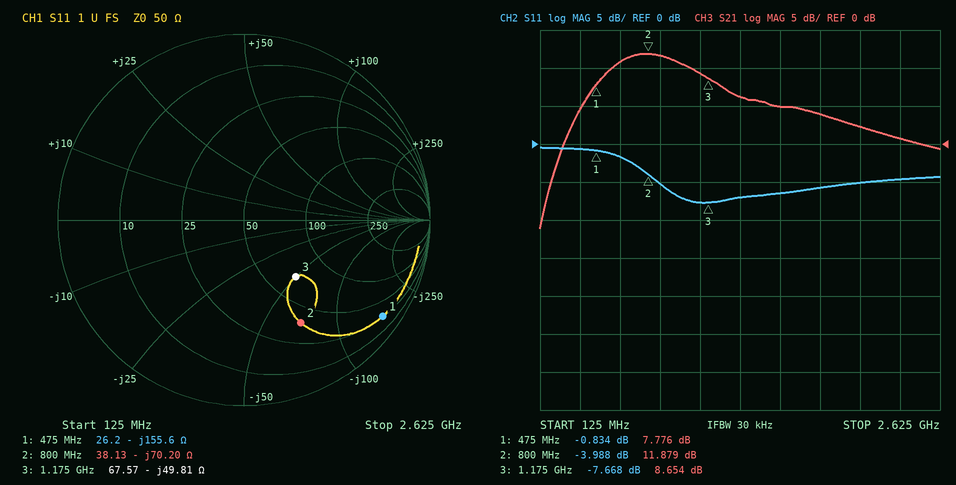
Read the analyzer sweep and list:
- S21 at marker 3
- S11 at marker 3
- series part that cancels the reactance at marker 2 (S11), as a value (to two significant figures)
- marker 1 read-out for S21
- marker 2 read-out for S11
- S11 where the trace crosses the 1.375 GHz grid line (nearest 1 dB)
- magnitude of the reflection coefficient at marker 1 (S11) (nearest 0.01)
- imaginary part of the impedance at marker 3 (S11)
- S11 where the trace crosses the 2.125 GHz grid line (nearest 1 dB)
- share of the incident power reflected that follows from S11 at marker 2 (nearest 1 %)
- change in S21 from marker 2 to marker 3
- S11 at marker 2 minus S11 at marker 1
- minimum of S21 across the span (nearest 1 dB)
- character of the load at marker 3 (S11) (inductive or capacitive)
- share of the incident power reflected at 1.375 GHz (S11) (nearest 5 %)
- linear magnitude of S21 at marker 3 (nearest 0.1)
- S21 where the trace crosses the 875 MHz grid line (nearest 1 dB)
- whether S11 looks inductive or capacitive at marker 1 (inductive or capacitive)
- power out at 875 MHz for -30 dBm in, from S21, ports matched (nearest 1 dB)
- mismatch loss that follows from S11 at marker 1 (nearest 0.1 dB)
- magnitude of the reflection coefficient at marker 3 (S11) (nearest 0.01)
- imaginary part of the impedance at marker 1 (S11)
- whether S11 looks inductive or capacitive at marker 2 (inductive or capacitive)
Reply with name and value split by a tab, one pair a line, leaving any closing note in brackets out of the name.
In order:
S21 at marker 3	8.654 dB
S11 at marker 3	-7.668 dB
series part that cancels the reactance at marker 2 (S11), as a value	14 nH
marker 1 read-out for S21	7.776 dB
marker 2 read-out for S11	-3.988 dB
S11 where the trace crosses the 1.375 GHz grid line	-7 dB
magnitude of the reflection coefficient at marker 1 (S11)	0.91
imaginary part of the impedance at marker 3	-49.81 Ω
S11 where the trace crosses the 2.125 GHz grid line	-5 dB
share of the incident power reflected that follows from S11 at marker 2	40 %
change in S21 from marker 2 to marker 3	-3.225 dB
S11 at marker 2 minus S11 at marker 1	-3.154 dB
minimum of S21 across the span	-11 dB
character of the load at marker 3 (S11)	capacitive
share of the incident power reflected at 1.375 GHz (S11)	20 %
linear magnitude of S21 at marker 3	2.7
S21 where the trace crosses the 875 MHz grid line	12 dB
whether S11 looks inductive or capacitive at marker 1	capacitive
power out at 875 MHz for -30 dBm in, from S21, ports matched	-18 dBm
mismatch loss that follows from S11 at marker 1	7.6 dB
magnitude of the reflection coefficient at marker 3 (S11)	0.41
imaginary part of the impedance at marker 1	-155.6 Ω
whether S11 looks inductive or capacitive at marker 2	capacitive
